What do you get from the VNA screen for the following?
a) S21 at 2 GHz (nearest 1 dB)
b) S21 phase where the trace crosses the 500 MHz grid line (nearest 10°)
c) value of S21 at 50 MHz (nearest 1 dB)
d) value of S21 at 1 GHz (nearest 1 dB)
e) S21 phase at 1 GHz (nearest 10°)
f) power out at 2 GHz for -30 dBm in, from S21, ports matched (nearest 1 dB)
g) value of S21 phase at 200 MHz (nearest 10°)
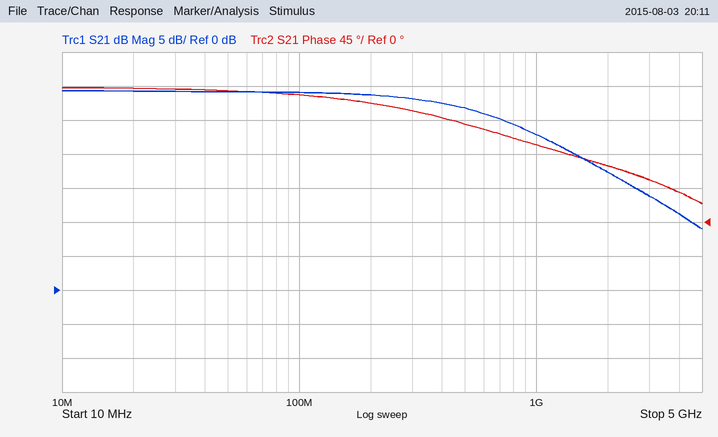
17 dB
130°
29 dB
23 dB
100°
-13 dBm
160°
